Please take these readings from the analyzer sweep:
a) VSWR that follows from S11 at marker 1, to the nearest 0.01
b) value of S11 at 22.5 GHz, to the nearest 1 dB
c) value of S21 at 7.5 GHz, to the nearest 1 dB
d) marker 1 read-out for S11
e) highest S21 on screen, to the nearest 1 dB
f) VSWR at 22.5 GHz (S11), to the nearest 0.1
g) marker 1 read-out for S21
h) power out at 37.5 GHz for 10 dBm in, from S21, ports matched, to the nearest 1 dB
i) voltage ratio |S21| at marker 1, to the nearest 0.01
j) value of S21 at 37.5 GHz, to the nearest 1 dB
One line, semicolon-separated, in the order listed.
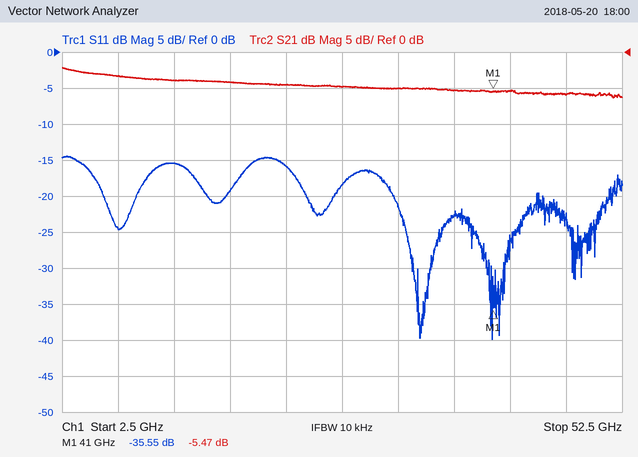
1.03; -16 dB; -3 dB; -35.55 dB; -2 dB; 1.4; -5.47 dB; 5 dBm; 0.53; -5 dB
